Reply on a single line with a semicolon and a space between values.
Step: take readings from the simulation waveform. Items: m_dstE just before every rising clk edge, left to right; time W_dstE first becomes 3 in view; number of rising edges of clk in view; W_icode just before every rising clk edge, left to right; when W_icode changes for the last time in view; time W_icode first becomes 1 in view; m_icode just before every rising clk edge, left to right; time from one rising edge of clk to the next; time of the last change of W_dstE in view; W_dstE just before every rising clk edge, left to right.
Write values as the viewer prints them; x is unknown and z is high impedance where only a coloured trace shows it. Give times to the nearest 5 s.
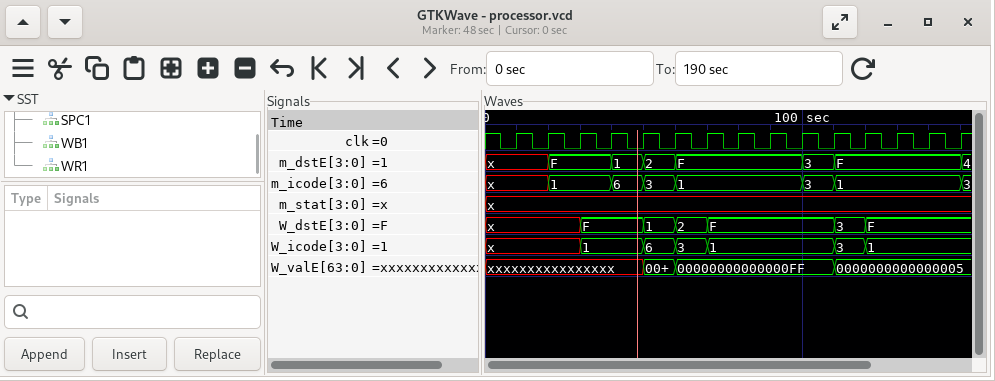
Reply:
x, x, F, F, 1, 2, F, F, F, F, 3, F, F, F, F; 110 s; 15; x, x, x, 1, 1, 6, 3, 1, 1, 1, 1, 3, 1, 1, 1; 120 s; 30 s; x, x, 1, 1, 6, 3, 1, 1, 1, 1, 3, 1, 1, 1, 1; 10 s; 120 s; x, x, x, F, F, 1, 2, F, F, F, F, 3, F, F, F
